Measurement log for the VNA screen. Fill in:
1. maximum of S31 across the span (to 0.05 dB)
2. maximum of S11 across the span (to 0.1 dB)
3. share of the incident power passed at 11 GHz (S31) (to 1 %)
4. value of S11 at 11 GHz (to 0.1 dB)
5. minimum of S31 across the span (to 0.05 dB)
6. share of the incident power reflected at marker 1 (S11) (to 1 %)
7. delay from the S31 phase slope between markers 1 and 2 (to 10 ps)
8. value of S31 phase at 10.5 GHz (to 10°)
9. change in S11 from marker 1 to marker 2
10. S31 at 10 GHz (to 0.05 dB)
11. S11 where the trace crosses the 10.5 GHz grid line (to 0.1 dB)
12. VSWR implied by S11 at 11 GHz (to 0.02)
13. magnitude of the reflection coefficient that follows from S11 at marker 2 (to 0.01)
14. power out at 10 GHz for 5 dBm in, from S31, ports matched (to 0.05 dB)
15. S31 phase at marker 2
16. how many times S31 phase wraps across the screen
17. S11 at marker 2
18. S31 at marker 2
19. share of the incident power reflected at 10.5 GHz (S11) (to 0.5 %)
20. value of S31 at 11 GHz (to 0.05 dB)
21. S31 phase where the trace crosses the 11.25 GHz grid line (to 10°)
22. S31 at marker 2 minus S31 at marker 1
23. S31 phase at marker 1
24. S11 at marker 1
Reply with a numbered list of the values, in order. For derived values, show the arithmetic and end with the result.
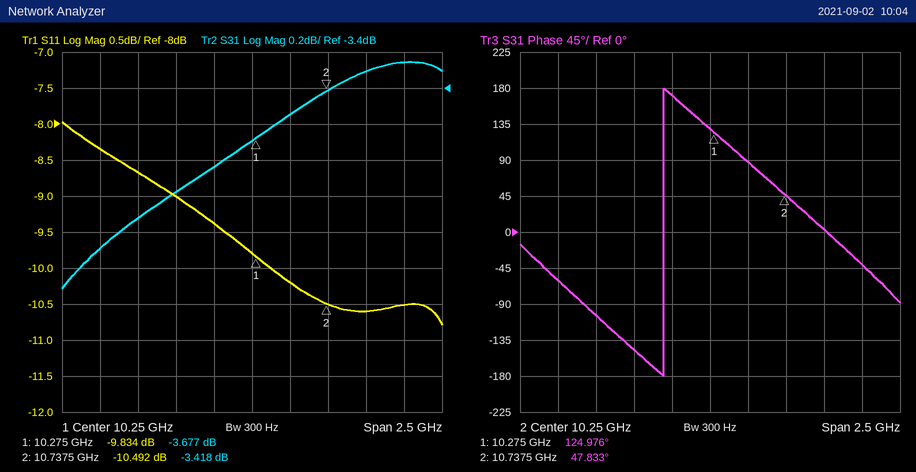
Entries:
1. -3.25 dB
2. -8.0 dB
3. 10^(-3.3/10) ≈ 47 %
4. -10.6 dB
5. -4.50 dB
6. 10^(-9.834/10) ≈ 10 %
7. −(47.833° − (124.976°))/(360° × 462.5 MHz) ≈ 463 ps, so 460 ps to the nearest 10 ps
8. 90°
9. -10.492 − (-9.834) = -0.658 dB
10. -3.85 dB
11. -10.2 dB
12. |Γ| = 10^(-10.6/20) = 0.2951; VSWR = (1 + 0.2951)/(1 − 0.2951) ≈ 1.84
13. 10^(-10.492/20) ≈ 0.30
14. 5 dBm + (-3.85 dB) = 1.15 dBm
15. 47.833°
16. 1
17. -10.492 dB
18. -3.418 dB
19. 10^(-10.2/10) ≈ 9.5 %
20. -3.30 dB
21. -40°
22. -3.418 − (-3.677) = 0.259 dB
23. 124.976°
24. -9.834 dB
